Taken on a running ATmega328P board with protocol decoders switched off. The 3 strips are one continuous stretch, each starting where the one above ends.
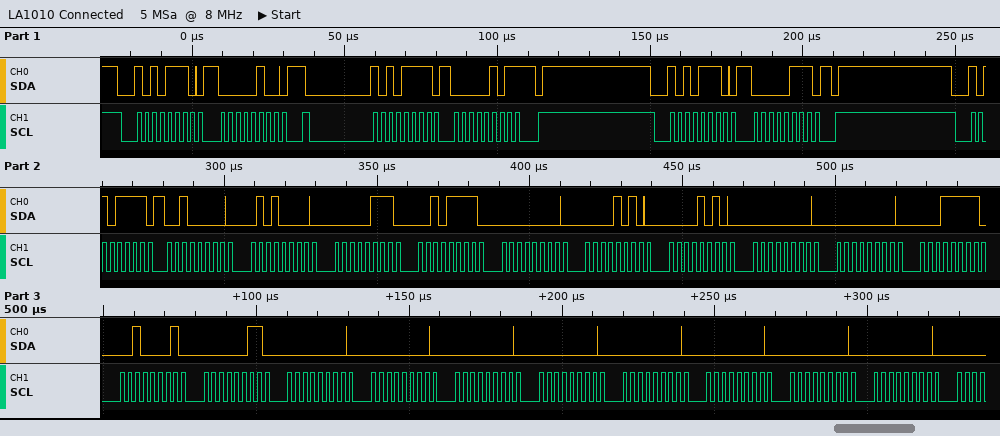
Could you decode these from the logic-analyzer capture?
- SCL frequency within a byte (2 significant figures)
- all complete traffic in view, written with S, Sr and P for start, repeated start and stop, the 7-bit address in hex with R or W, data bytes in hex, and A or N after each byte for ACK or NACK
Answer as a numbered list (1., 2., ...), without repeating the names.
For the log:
1. 400 kHz
2. S 57W A 04 A Sr 57R A 05 N P S 57W A 07 A P S 57R A 20 A 50 A 07 A 2F A 00 A 0A A 0A A 00 A 00 A 1F A 21 A 03 A 00 A 00 A 00 A 00 A 00 A 00 A 00 A 00 A
